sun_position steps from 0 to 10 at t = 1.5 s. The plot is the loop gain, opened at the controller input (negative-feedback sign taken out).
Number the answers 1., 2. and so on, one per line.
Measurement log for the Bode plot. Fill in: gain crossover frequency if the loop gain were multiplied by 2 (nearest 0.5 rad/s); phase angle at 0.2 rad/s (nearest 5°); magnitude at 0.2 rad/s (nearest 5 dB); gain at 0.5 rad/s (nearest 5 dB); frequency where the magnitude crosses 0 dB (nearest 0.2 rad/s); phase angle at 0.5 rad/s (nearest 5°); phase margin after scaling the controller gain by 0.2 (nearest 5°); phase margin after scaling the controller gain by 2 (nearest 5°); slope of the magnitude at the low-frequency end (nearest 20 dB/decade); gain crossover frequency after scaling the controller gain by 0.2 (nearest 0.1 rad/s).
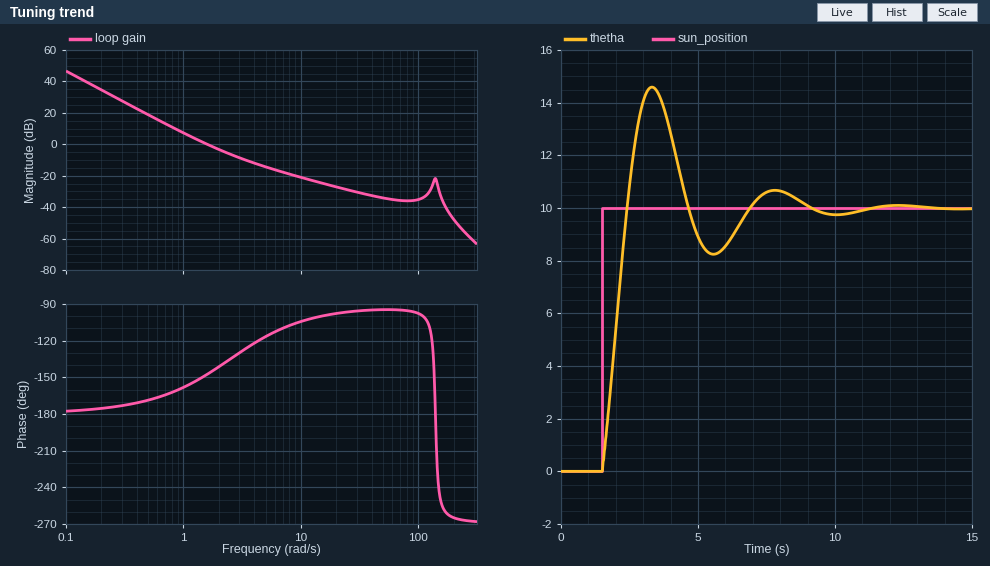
1. 2.5 rad/s
2. -175°
3. 35 dB
4. 20 dB
5. 1.6 rad/s
6. -170°
7. 15°
8. 45°
9. -40 dB/decade
10. 0.7 rad/s
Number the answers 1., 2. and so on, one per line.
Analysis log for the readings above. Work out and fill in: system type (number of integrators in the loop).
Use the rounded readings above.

1. 2
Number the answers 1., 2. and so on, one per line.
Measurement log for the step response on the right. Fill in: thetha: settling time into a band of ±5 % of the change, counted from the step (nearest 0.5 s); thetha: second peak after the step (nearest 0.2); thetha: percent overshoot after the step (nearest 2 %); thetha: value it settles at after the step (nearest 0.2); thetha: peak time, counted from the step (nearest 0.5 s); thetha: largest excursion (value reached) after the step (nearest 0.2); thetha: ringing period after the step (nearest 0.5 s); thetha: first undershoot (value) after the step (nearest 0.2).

1. 7.0 s
2. 10.6
3. 46 %
4. 10.0
5. 2.0 s
6. 14.6
7. 4.5 s
8. 8.2
